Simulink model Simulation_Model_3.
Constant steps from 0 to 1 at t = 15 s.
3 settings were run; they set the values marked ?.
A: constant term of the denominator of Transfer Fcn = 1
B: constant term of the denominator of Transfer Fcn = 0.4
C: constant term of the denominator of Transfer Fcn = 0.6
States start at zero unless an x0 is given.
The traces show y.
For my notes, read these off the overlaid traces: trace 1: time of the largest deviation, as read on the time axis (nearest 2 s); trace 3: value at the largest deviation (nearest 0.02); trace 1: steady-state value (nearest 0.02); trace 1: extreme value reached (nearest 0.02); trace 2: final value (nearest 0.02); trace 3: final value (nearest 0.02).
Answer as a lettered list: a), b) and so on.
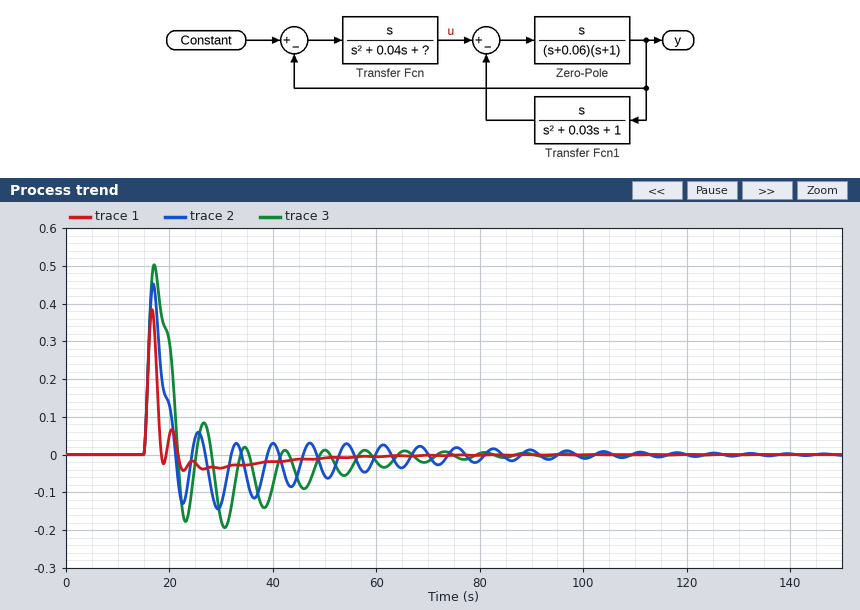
a) 16 s
b) 0.50
c) 0.00
d) 0.38
e) 0.00
f) 0.00
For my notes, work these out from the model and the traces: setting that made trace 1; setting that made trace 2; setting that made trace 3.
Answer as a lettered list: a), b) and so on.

a) A
b) C
c) B
